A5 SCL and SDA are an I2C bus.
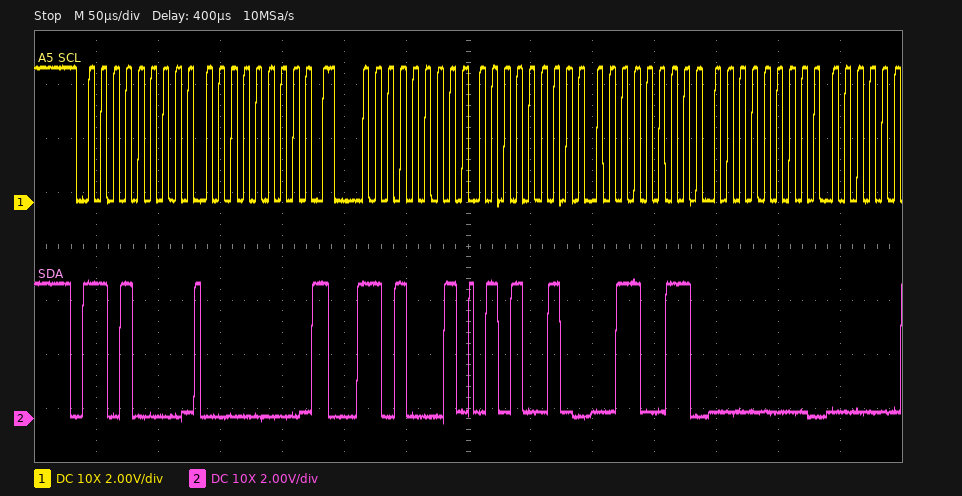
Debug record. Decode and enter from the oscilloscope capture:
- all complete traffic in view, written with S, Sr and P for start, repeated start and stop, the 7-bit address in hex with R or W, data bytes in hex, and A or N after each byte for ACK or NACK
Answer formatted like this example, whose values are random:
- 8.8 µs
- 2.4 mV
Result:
- S 68W A 00 A Sr 68R A 52 A 33 A 00 A
